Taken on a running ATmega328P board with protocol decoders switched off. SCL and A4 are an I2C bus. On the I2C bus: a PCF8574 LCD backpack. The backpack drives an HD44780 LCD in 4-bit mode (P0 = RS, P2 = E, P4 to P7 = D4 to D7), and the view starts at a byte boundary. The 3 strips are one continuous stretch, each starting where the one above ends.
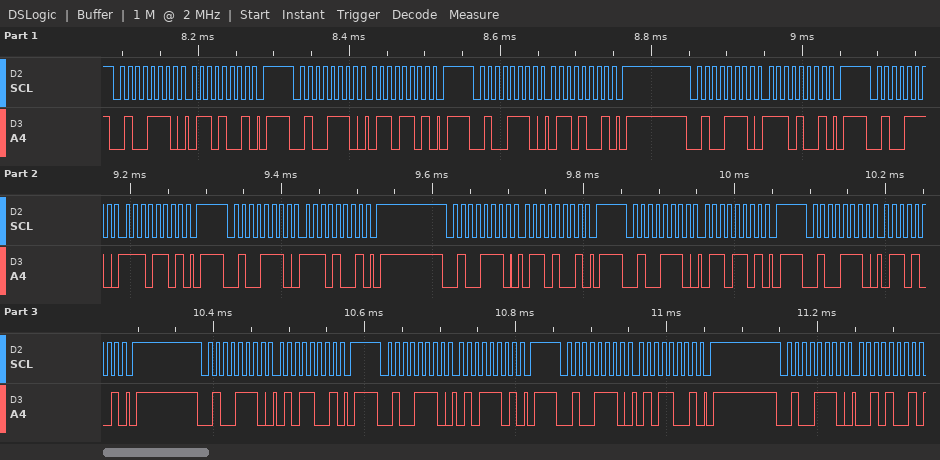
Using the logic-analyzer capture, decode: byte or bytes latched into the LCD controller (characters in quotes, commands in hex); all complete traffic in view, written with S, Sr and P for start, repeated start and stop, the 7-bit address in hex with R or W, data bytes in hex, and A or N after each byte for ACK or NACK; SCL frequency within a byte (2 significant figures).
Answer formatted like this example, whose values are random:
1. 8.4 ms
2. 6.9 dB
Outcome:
1. 'n' 'e'
2. S 27W A 69 A P S 27W A 6D A P S 27W A 69 A P S 27W A E9 A P S 27W A ED A P S 27W A E9 A P S 27W A 69 A P S 27W A 6D A P S 27W A 69 A P S 27W A 59 A P S 27W A 5D A P S 27W A 59 A P S 27W A 29 A
3. 100 kHz
